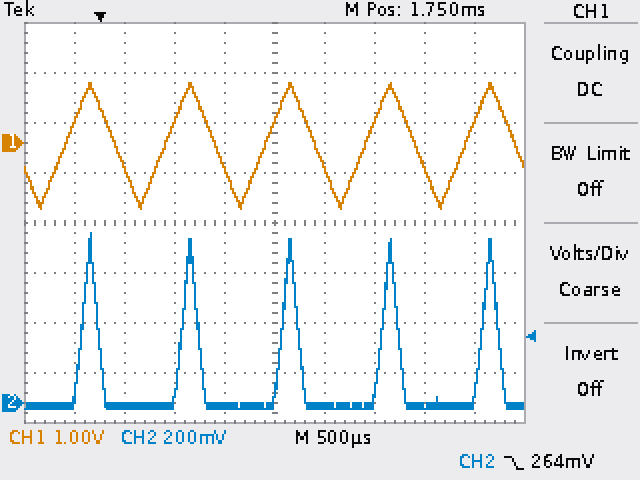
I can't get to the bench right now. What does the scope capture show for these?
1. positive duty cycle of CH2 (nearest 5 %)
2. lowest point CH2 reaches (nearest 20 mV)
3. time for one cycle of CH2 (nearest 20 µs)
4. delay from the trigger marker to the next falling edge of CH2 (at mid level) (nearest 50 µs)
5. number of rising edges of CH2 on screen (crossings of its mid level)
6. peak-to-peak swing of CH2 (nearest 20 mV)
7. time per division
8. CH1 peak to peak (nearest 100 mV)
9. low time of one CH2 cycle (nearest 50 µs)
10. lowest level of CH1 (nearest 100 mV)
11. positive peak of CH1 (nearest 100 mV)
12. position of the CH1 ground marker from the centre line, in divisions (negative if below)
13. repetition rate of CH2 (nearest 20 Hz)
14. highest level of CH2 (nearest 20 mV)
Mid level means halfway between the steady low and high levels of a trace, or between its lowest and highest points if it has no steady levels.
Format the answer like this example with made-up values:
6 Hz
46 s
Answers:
15 %
-20 mV
1.00 ms
1.00 ms
5
700 mV
500 µs
2.5 V
850 µs
-1.3 V
1.2 V
+1.6 div
1.00 kHz
680 mV
